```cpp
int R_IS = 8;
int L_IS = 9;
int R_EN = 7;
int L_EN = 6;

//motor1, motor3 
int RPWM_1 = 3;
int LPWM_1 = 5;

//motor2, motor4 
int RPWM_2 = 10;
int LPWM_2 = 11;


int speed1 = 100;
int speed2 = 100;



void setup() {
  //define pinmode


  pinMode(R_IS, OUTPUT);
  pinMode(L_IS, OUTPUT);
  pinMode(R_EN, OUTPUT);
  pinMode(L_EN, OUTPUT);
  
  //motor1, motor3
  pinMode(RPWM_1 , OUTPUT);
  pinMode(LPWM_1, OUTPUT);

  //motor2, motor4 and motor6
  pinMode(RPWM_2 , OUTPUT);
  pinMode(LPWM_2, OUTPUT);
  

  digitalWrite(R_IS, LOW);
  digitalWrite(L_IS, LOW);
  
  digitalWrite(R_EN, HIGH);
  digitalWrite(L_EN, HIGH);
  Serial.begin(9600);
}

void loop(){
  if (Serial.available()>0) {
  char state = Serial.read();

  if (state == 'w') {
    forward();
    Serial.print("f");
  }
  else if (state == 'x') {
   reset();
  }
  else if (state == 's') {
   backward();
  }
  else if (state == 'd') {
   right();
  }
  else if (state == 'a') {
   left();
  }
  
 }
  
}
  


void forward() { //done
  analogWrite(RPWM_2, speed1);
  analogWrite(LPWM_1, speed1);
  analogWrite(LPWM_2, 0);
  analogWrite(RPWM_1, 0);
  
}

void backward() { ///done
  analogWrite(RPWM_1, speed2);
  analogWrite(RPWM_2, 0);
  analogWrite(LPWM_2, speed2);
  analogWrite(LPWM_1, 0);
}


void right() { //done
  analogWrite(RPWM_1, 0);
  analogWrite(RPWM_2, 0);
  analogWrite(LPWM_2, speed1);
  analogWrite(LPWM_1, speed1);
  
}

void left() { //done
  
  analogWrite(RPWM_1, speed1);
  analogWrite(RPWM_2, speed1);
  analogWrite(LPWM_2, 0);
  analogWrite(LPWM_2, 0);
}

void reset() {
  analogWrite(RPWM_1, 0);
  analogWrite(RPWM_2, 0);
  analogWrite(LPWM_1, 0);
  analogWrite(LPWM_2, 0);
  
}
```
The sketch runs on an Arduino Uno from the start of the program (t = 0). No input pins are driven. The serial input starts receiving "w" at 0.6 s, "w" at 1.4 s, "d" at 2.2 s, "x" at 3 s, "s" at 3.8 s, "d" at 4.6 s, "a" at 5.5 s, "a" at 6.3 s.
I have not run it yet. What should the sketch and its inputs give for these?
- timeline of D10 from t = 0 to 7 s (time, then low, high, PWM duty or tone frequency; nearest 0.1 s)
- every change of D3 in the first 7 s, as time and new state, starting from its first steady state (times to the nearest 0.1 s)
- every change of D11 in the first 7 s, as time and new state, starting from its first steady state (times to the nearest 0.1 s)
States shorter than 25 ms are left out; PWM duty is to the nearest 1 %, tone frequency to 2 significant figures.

0 s low; 0.6 s PWM 39 %; 2.2 s low; 5.5 s PWM 39 %
0 s low; 3.8 s PWM 39 %; 4.6 s low; 5.5 s PWM 39 %
0 s low; 2.2 s PWM 39 %; 3 s low; 3.8 s PWM 39 %; 5.5 s low
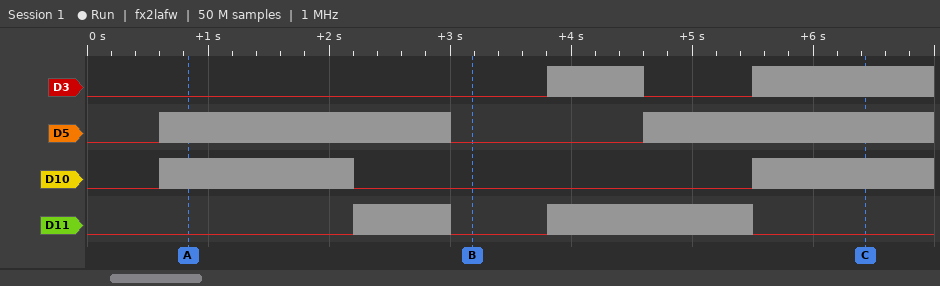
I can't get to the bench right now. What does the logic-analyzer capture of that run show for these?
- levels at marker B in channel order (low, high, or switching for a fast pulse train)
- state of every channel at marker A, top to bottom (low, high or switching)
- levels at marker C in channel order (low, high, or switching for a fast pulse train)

D3 low, D5 low, D10 low, D11 low
D3 low, D5 switching, D10 switching, D11 low
D3 switching, D5 switching, D10 switching, D11 low
